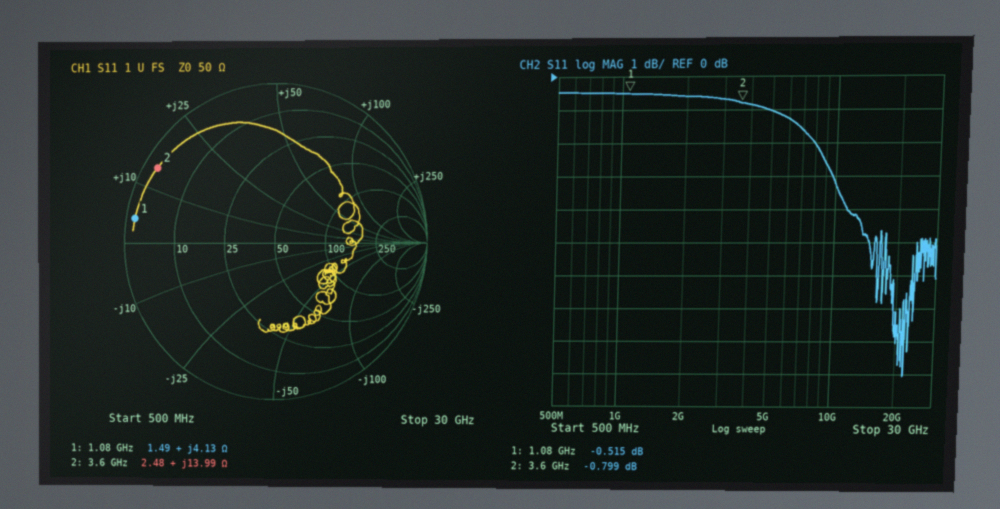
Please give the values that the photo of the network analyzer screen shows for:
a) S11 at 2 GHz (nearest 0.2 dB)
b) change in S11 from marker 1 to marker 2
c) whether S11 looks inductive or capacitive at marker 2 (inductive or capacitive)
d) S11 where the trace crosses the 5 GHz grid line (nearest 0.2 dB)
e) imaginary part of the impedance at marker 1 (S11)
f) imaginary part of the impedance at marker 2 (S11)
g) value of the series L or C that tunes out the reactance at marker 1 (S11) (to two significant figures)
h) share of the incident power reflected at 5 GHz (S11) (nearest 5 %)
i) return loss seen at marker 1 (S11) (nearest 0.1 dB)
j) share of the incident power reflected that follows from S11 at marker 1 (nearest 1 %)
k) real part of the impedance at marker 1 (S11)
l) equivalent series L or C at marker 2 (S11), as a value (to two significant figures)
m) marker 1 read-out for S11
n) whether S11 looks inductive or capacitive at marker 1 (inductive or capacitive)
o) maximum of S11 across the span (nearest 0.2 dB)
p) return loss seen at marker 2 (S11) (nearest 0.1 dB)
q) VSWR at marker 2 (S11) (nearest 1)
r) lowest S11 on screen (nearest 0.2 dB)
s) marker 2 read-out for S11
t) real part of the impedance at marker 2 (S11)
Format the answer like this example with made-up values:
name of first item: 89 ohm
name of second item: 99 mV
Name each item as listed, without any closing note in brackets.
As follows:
S11 at 2 GHz: -0.6 dB
change in S11 from marker 1 to marker 2: -0.284 dB
whether S11 looks inductive or capacitive at marker 2: inductive
S11 where the trace crosses the 5 GHz grid line: -1.0 dB
imaginary part of the impedance at marker 1: +4.13 Ω
imaginary part of the impedance at marker 2: +13.99 Ω
value of the series L or C that tunes out the reactance at marker 1 (S11): 36 pF
share of the incident power reflected at 5 GHz (S11): 80 %
return loss seen at marker 1 (S11): 0.5 dB
share of the incident power reflected that follows from S11 at marker 1: 89 %
real part of the impedance at marker 1: 1.49 Ω
equivalent series L or C at marker 2 (S11), as a value: 620 pH
marker 1 read-out for S11: -0.515 dB
whether S11 looks inductive or capacitive at marker 1: inductive
maximum of S11 across the span: -0.4 dB
return loss seen at marker 2 (S11): 0.8 dB
VSWR at marker 2 (S11): 22
lowest S11 on screen: -9.0 dB
marker 2 read-out for S11: -0.799 dB
real part of the impedance at marker 2: 2.48 Ω
